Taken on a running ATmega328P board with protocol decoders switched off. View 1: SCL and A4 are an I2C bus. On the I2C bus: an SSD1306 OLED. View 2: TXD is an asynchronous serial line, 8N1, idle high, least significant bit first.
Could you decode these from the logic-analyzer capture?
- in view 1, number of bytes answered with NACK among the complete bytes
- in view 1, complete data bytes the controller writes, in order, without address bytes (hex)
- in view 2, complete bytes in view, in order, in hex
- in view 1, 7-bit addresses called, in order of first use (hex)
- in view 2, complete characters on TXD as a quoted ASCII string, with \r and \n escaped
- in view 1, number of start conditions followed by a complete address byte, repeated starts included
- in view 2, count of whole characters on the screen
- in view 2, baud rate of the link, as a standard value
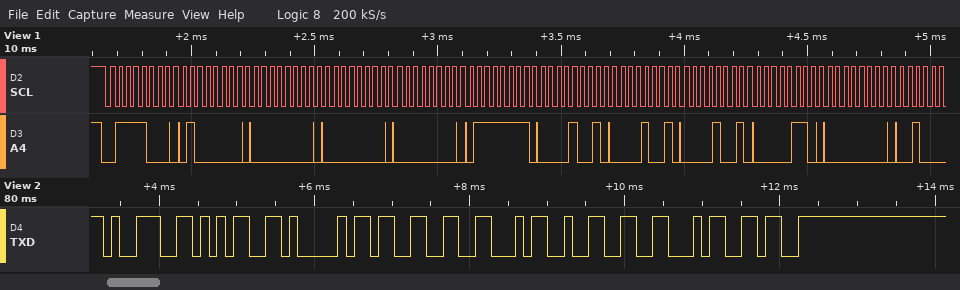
0
40 00 00 00 7F 09 09 09 06 00
39 35 41 33 46 32 46 36
0x3C
"95A3F2F6"
1
8
9600 baud
